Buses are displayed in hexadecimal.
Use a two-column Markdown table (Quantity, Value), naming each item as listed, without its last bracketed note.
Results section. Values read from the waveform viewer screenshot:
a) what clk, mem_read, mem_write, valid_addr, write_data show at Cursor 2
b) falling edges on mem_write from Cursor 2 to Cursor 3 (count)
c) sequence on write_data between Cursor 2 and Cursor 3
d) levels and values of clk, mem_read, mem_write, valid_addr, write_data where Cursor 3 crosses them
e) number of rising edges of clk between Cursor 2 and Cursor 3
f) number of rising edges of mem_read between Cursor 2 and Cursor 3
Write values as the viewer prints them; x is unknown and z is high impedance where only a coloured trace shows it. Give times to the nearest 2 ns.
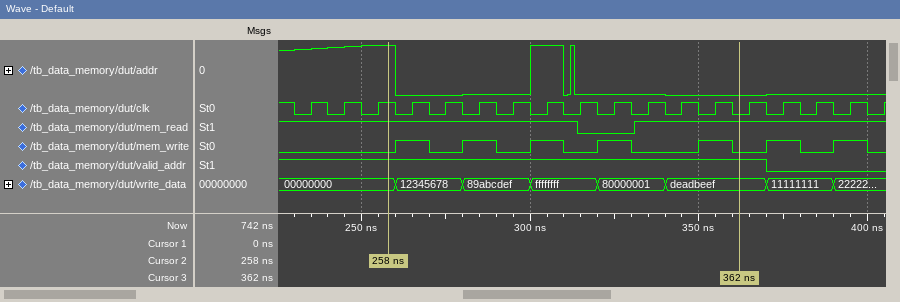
| Quantity | Value |
|---|---|
| what clk, mem_read, mem_write, valid_addr, write_data show at Cursor 2 | clk=1, mem_read=1, mem_write=0, valid_addr=1, write_data=00000000 |
| falling edges on mem_write from Cursor 2 to Cursor 3 | 5 |
| sequence on write_data between Cursor 2 and Cursor 3 | 00000000, 12345678, 89abcdef, ffffffff, 80000001, deadbeef |
| levels and values of clk, mem_read, mem_write, valid_addr, write_data where Cursor 3 crosses them | clk=0, mem_read=1, mem_write=0, valid_addr=1, write_data=deadbeef |
| number of rising edges of clk between Cursor 2 and Cursor 3 | 10 |
| number of rising edges of mem_read between Cursor 2 and Cursor 3 | 1 |
